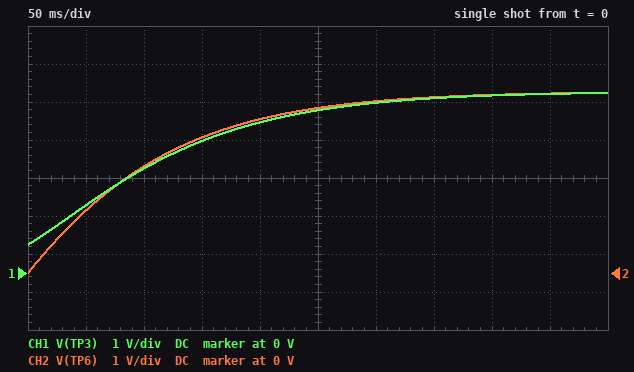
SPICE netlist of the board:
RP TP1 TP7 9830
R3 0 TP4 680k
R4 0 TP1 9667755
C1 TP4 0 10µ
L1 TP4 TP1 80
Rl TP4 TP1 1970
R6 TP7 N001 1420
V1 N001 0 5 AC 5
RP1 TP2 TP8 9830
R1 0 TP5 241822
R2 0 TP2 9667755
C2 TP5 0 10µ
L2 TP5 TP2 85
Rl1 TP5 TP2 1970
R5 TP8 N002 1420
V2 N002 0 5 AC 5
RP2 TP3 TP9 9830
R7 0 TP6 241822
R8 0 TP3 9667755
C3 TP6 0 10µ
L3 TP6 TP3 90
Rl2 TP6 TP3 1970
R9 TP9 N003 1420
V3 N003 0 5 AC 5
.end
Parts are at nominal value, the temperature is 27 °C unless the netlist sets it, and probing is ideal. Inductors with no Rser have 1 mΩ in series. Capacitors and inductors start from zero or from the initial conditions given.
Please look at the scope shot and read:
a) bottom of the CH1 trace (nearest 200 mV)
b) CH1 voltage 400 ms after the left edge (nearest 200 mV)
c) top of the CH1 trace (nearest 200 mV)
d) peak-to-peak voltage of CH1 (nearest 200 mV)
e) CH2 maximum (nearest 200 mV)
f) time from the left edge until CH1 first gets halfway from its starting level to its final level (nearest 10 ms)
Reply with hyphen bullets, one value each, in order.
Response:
- 800 mV
- 4.6 V
- 4.8 V
- 4.0 V
- 4.8 V
- 100 ms
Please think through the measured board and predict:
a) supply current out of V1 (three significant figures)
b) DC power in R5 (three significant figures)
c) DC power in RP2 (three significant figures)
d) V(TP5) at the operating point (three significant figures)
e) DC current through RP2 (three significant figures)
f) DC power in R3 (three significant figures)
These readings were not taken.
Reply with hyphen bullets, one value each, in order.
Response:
- 7.73 µA
- 581 nW
- 4.02 µW
- 4.77 V
- 20.2 µA
- 35.5 µW
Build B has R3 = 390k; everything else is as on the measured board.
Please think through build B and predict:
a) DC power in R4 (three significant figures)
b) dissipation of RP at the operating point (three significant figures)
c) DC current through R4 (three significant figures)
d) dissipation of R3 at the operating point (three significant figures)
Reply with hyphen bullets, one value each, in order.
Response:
- 2.44 µW
- 1.65 µW
- 502 nA
- 60.4 µW
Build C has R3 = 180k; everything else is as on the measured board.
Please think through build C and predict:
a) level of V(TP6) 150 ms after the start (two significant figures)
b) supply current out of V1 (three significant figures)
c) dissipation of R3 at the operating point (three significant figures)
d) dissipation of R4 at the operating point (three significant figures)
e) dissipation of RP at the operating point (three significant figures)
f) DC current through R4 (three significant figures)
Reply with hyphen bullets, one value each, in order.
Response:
- 3.6 V
- 26.6 µA
- 123 µW
- 2.29 µW
- 6.96 µW
- 486 nA
